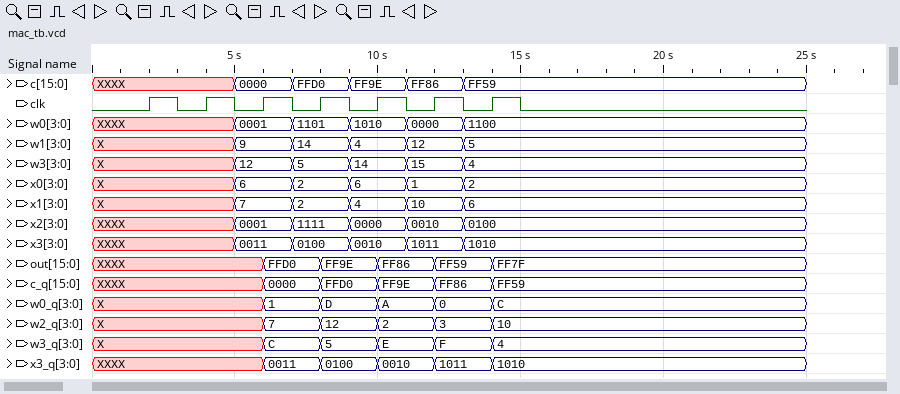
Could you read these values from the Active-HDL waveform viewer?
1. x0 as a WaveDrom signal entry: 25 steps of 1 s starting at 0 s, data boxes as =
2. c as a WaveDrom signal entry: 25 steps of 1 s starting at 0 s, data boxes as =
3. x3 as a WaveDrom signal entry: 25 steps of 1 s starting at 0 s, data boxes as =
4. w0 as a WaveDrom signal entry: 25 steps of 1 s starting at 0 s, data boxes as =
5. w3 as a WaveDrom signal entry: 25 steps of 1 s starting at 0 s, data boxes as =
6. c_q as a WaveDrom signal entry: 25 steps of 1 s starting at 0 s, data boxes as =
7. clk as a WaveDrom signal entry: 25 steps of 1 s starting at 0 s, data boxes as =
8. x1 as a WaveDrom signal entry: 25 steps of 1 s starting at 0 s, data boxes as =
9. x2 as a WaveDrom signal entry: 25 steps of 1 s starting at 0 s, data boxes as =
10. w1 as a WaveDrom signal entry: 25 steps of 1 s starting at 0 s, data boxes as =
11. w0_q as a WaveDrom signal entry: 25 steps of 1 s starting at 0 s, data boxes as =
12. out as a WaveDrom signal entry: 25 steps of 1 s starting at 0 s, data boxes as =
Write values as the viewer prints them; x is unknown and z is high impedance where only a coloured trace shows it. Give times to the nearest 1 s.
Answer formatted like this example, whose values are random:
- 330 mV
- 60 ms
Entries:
- {name: 'x0', wave: 'x....=.=.=.=.=...........', data: '6 2 6 1 2'}
- {name: 'c', wave: 'x....=.=.=.=.=...........', data: '0000 FFD0 FF9E FF86 FF59'}
- {name: 'x3', wave: 'x....=.=.=.=.=...........', data: '0011 0100 0010 1011 1010'}
- {name: 'w0', wave: 'x....=.=.=.=.=...........', data: '0001 1101 1010 0000 1100'}
- {name: 'w3', wave: 'x....=.=.=.=.=...........', data: '12 5 14 15 4'}
- {name: 'c_q', wave: 'x.....=.=.=.=.=..........', data: '0000 FFD0 FF9E FF86 FF59'}
- {name: 'clk', wave: '0.10101010101010.........'}
- {name: 'x1', wave: 'x....=.=.=.=.=...........', data: '7 2 4 10 6'}
- {name: 'x2', wave: 'x....=.=.=.=.=...........', data: '0001 1111 0000 0010 0100'}
- {name: 'w1', wave: 'x....=.=.=.=.=...........', data: '9 14 4 12 5'}
- {name: 'w0_q', wave: 'x.....=.=.=.=.=..........', data: '1 D A 0 C'}
- {name: 'out', wave: 'x.....=.=.=.=.=..........', data: 'FFD0 FF9E FF86 FF59 FF7F'}
